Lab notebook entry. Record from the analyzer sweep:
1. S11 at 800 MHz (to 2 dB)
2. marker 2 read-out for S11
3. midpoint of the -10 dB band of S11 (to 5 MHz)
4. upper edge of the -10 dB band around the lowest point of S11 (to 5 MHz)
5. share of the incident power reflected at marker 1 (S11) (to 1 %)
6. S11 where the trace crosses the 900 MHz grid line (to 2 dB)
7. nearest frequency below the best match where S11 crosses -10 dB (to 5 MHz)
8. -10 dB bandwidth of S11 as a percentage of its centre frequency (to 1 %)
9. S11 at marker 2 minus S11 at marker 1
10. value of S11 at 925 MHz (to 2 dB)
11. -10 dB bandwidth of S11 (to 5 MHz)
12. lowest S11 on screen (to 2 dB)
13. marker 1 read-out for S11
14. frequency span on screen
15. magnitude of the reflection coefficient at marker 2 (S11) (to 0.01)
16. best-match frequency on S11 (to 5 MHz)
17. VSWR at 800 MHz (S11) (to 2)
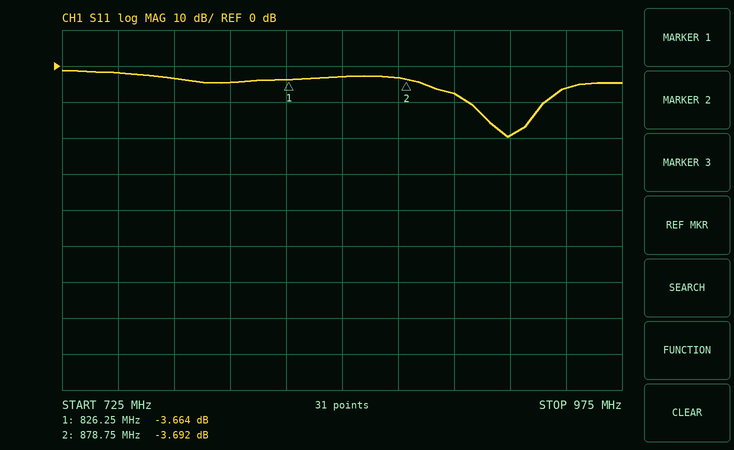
-4 dB
-3.692 dB
925 MHz
940 MHz
43 %
-8 dB
905 MHz
4 %
-0.028 dB
-20 dB
35 MHz
-20 dB
-3.664 dB
250 MHz
0.65
925 MHz
4
